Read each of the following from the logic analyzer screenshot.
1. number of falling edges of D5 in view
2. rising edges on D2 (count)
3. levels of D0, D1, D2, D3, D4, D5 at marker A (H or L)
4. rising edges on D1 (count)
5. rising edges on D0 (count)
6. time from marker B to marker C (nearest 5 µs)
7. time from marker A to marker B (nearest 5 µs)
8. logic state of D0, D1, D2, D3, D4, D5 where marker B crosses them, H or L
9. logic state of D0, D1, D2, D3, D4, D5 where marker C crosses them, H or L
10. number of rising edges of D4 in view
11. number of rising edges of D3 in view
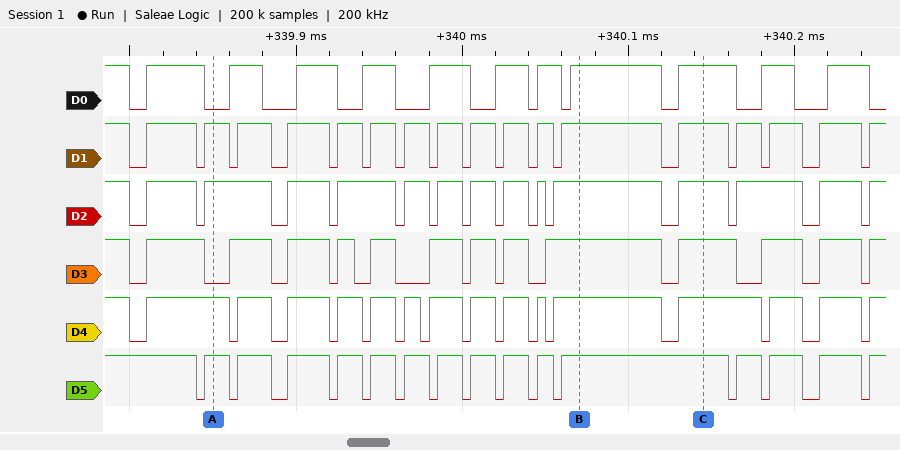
15
14
D0=L, D1=H, D2=H, D3=L, D4=H, D5=H
17
11
75 µs
220 µs
D0=H, D1=H, D2=H, D3=H, D4=H, D5=H
D0=H, D1=H, D2=H, D3=H, D4=H, D5=H
15
13
